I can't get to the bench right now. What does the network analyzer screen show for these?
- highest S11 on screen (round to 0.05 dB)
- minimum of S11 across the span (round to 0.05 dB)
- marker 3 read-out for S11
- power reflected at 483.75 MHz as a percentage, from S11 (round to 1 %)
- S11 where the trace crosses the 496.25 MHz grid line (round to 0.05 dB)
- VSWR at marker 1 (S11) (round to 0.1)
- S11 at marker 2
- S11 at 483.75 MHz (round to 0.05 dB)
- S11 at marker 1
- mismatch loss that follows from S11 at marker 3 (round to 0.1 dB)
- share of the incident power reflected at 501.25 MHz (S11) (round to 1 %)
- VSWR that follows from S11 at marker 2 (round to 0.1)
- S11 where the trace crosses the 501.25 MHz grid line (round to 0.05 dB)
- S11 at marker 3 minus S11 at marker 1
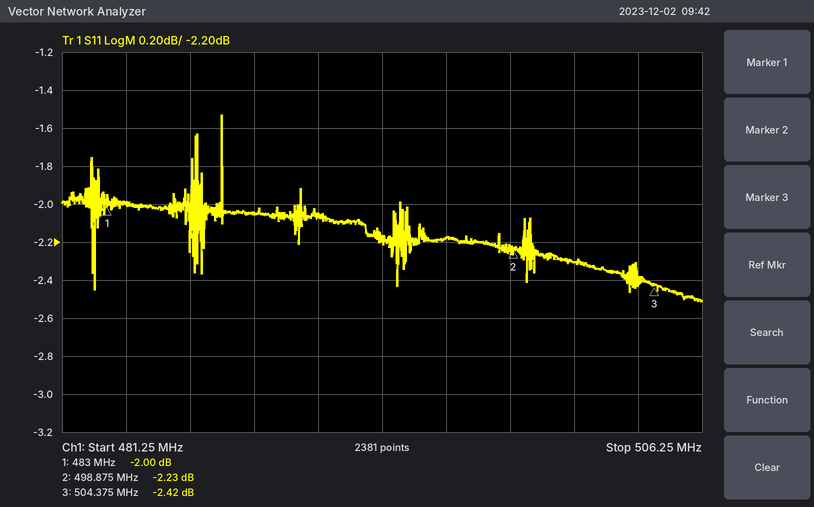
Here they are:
-1.55 dB
-2.50 dB
-2.42 dB
63 %
-2.20 dB
8.7
-2.23 dB
-2.00 dB
-2.00 dB
3.7 dB
59 %
7.8
-2.30 dB
-0.42 dB
